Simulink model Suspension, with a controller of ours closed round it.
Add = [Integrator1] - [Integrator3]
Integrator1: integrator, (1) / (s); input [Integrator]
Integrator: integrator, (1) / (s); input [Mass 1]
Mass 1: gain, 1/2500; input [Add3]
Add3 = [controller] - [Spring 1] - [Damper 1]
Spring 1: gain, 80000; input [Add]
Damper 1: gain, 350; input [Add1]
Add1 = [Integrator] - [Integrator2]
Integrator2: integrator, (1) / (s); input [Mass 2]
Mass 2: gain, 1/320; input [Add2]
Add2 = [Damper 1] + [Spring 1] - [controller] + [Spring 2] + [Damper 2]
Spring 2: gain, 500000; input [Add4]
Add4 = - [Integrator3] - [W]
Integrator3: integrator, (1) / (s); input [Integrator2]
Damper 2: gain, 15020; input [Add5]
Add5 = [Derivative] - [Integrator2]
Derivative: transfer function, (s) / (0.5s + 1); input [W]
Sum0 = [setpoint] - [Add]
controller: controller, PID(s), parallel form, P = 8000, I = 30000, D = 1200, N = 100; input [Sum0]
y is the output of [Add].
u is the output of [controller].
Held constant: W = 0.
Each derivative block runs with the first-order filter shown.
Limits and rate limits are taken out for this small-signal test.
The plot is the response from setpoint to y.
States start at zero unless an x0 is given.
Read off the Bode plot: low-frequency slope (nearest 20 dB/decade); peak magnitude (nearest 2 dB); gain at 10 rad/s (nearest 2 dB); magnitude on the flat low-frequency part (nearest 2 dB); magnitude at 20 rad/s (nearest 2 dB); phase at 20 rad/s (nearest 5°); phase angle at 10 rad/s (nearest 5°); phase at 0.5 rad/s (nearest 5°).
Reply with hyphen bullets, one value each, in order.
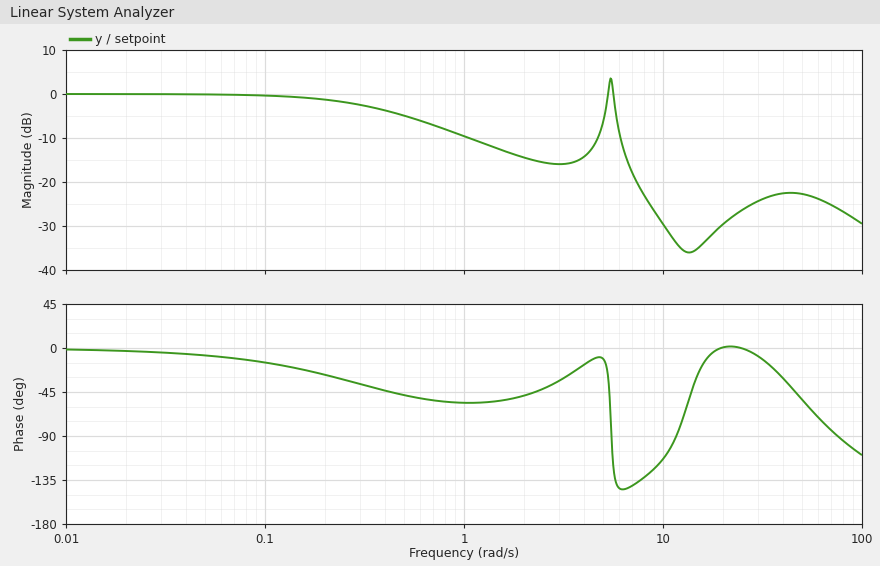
- 0 dB/decade
- 4 dB
- -30 dB
- 0 dB
- -30 dB
- 0°
- -115°
- -50°
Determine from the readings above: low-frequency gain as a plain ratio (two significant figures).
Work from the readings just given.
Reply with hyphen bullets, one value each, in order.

- 1.0
